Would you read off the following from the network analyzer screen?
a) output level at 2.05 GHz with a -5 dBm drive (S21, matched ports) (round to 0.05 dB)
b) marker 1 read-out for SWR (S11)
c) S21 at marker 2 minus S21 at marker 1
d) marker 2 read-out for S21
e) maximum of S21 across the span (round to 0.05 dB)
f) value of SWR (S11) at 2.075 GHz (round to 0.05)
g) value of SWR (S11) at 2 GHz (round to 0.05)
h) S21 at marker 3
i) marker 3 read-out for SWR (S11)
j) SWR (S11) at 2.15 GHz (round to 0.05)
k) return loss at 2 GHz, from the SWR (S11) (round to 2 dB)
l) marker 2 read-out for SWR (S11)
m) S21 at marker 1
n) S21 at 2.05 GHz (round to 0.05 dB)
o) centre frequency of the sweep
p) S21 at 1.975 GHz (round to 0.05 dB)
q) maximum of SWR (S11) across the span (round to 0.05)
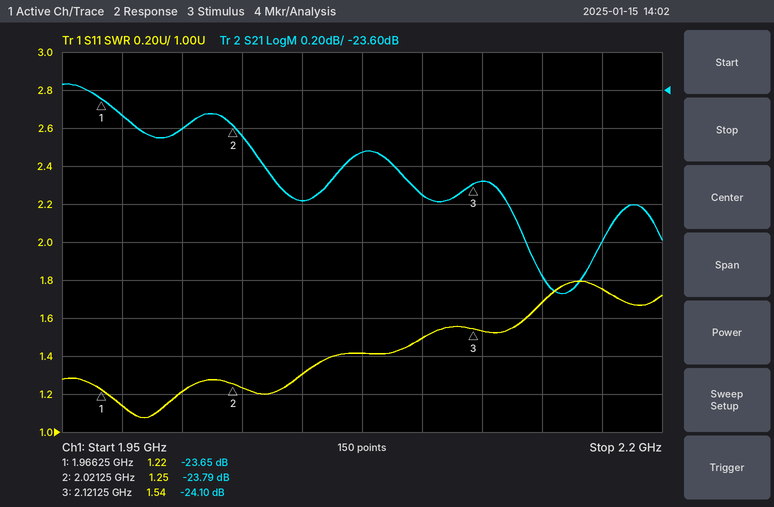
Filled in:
-29.20 dBm
1.22
-0.14 dB
-23.79 dB
-23.55 dB
1.40
1.20
-24.10 dB
1.54
1.70
20 dB
1.25
-23.65 dB
-24.20 dB
2.075 GHz
-23.75 dB
1.80
